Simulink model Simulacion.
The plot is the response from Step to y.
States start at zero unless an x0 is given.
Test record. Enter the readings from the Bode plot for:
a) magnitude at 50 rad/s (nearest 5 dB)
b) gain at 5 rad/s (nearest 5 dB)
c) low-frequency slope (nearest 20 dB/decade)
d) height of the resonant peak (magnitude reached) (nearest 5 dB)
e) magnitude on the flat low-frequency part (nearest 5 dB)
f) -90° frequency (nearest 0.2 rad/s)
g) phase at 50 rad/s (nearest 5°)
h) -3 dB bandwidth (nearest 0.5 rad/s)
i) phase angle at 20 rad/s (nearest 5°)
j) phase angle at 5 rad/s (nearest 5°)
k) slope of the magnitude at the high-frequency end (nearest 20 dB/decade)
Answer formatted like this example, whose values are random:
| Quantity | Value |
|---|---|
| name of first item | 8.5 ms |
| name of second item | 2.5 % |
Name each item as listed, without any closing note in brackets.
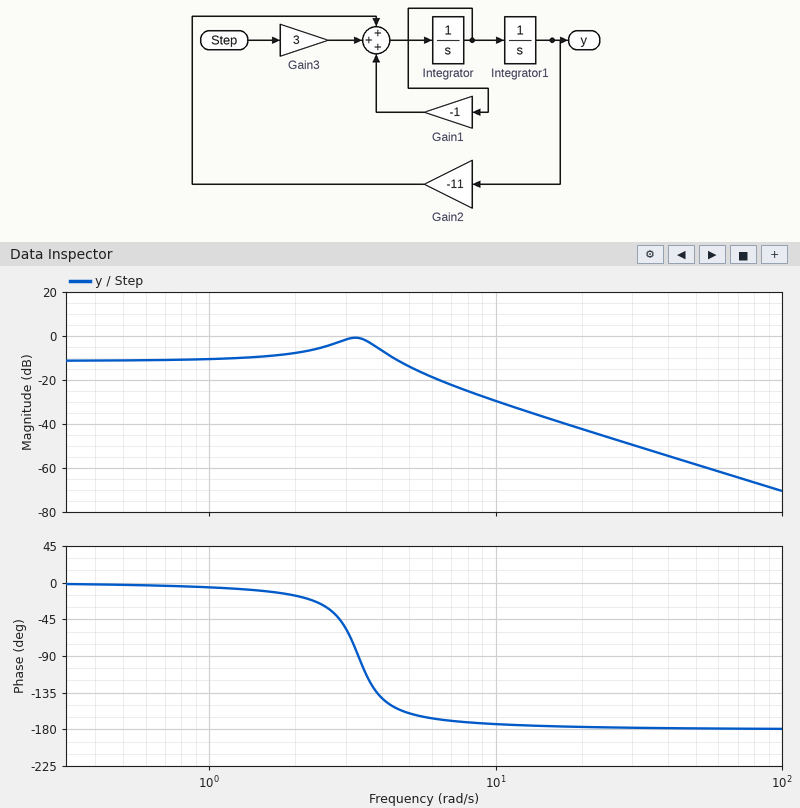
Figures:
| Quantity | Value |
|---|---|
| magnitude at 50 rad/s | -60 dB |
| gain at 5 rad/s | -15 dB |
| low-frequency slope | 0 dB/decade |
| height of the resonant peak (magnitude reached) | 0 dB |
| magnitude on the flat low-frequency part | -10 dB |
| -90° frequency | 3.4 rad/s |
| phase at 50 rad/s | -180° |
| -3 dB bandwidth | 5.0 rad/s |
| phase angle at 20 rad/s | -175° |
| phase angle at 5 rad/s | -160° |
| slope of the magnitude at the high-frequency end | -40 dB/decade |
